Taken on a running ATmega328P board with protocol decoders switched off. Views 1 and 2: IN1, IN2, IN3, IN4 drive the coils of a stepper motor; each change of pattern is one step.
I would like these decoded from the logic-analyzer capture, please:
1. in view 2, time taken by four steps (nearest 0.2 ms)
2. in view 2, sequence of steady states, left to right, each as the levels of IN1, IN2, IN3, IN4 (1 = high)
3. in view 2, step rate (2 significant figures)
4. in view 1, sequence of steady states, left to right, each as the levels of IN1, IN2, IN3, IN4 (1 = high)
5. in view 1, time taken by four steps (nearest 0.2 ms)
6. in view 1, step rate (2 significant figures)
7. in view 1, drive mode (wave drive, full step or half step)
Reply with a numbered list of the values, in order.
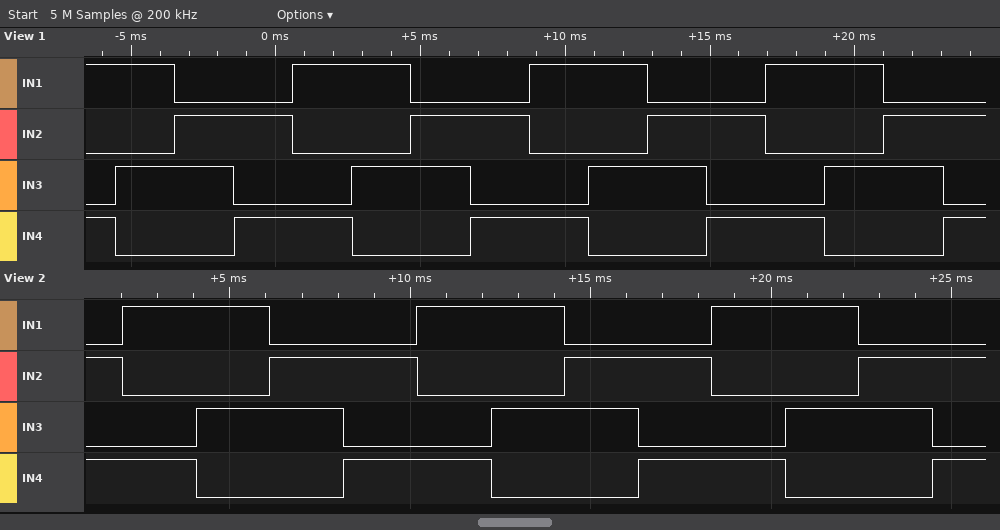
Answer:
1. 8.2 ms
2. 0101 1001 1010 0110 0101 1001 1010 0110 0101 1001 1010 0110 0101
3. 490 steps/s
4. 1001 1010 0110 0101 1001 1010 0110 0101 1001 1010 0110 0101 1001 1010 0110 0101
5. 8.2 ms
6. 490 steps/s
7. full step
